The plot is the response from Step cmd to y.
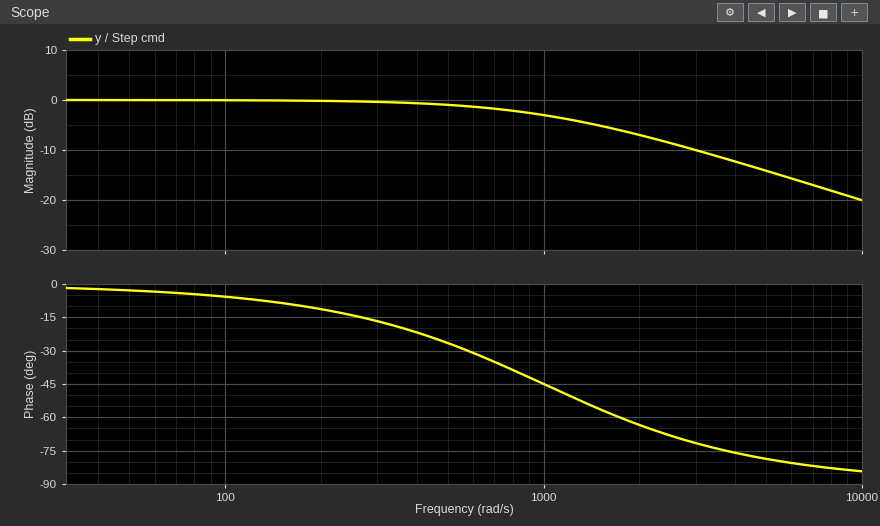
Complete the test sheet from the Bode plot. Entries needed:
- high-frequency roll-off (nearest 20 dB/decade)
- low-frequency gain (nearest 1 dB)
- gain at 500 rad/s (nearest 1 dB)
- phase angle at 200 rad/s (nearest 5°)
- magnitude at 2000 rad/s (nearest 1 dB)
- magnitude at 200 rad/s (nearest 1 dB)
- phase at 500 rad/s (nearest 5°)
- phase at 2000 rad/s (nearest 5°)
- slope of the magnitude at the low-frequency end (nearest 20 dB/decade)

-20 dB/decade
0 dB
-1 dB
-10°
-7 dB
0 dB
-25°
-65°
0 dB/decade
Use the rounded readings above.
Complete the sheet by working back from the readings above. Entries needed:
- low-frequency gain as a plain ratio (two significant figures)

1.0
